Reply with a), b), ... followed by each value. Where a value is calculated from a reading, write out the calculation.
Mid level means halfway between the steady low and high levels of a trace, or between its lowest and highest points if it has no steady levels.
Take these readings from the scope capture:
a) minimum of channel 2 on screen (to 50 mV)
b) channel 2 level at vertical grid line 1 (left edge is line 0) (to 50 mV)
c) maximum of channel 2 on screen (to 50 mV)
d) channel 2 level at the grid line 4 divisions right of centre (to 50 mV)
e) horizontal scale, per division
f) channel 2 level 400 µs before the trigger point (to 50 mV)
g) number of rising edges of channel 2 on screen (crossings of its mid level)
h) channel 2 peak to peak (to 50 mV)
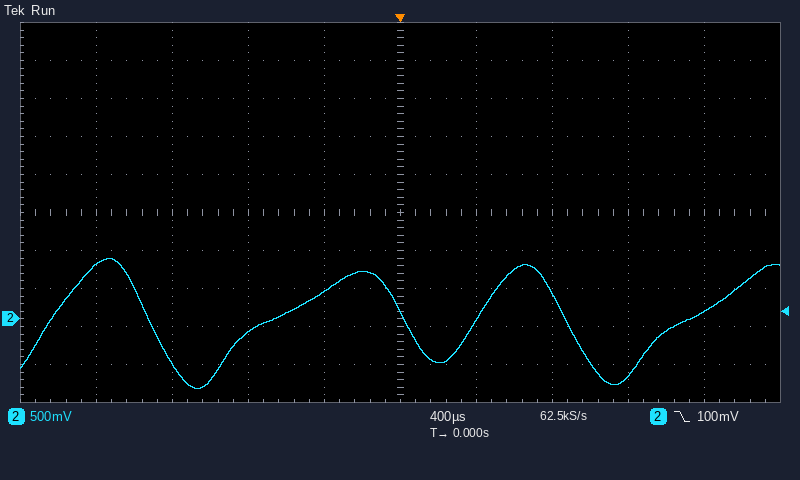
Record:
a) -900 mV
b) 700 mV
c) 800 mV
d) 100 mV
e) 400 µs
f) 350 mV
g) 4
h) 800 mV − (-900 mV) = 1.70 V
